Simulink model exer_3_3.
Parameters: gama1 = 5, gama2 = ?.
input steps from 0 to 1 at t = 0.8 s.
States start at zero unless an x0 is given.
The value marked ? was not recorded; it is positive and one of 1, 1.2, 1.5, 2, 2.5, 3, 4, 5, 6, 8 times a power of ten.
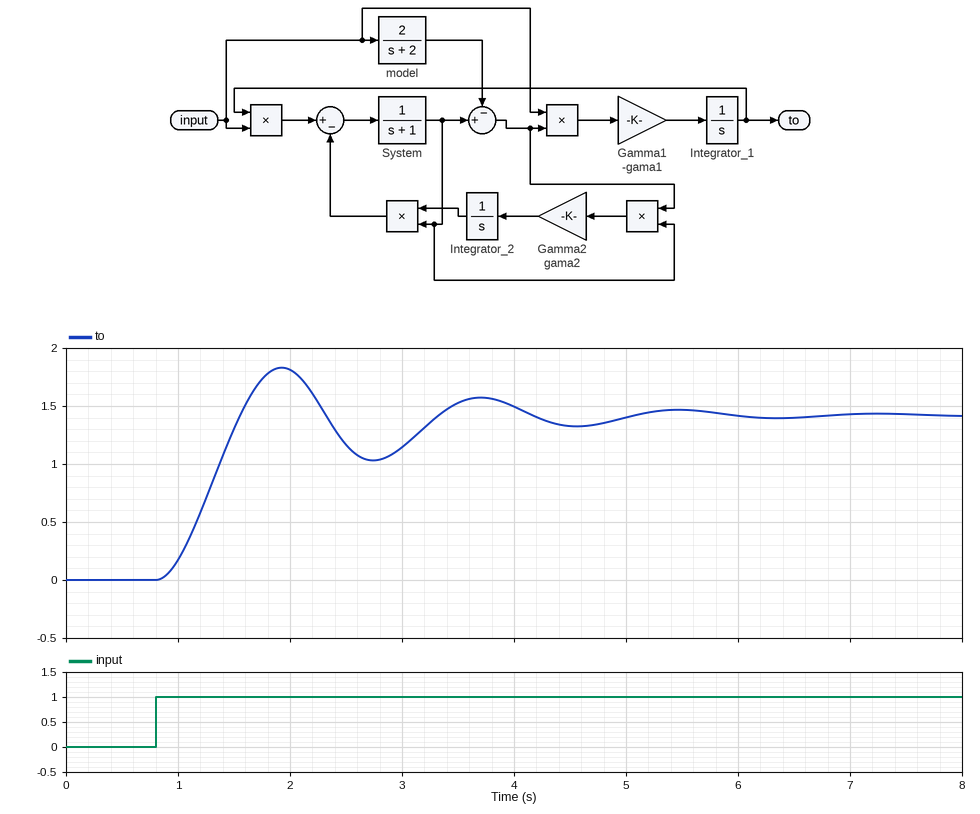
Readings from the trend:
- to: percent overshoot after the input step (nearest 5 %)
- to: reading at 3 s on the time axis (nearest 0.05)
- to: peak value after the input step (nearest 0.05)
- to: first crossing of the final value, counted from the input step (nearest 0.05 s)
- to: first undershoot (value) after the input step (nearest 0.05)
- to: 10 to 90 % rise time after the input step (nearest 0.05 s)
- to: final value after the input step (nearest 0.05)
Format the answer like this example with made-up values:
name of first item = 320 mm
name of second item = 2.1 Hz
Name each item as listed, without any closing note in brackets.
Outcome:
to: percent overshoot after the input step = 30 %
to: reading at 3 s on the time axis = 1.15
to: peak value after the input step = 1.85
to: first crossing of the final value, counted from the input step = 0.75 s
to: first undershoot (value) after the input step = 1.05
to: 10 to 90 % rise time after the input step = 0.50 s
to: final value after the input step = 1.40
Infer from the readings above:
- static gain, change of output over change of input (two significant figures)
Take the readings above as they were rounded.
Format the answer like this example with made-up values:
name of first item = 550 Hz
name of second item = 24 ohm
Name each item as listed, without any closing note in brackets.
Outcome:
static gain, change of output over change of input = 1.4
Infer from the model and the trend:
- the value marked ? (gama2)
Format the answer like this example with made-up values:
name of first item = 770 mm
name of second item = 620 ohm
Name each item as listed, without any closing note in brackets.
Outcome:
the value marked ? = 8
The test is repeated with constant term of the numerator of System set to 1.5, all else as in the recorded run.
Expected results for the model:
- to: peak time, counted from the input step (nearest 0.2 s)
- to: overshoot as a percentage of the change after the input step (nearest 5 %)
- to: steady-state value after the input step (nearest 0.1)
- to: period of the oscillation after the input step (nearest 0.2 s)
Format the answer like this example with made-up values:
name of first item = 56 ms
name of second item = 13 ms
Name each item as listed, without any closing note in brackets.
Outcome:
to: peak time, counted from the input step = 1.0 s
to: overshoot as a percentage of the change after the input step = 30 %
to: steady-state value after the input step = 1.0
to: period of the oscillation after the input step = 1.4 s
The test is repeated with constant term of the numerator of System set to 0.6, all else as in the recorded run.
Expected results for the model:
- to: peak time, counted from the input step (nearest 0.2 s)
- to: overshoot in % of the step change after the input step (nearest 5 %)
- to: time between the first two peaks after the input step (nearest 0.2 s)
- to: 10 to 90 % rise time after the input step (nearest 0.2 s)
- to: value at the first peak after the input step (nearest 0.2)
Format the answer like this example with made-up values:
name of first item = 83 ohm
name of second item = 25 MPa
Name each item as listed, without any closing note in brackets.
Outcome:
to: peak time, counted from the input step = 1.4 s
to: overshoot in % of the step change after the input step = 25 %
to: time between the first two peaks after the input step = 2.2 s
to: 10 to 90 % rise time after the input step = 0.6 s
to: value at the first peak after the input step = 2.6
